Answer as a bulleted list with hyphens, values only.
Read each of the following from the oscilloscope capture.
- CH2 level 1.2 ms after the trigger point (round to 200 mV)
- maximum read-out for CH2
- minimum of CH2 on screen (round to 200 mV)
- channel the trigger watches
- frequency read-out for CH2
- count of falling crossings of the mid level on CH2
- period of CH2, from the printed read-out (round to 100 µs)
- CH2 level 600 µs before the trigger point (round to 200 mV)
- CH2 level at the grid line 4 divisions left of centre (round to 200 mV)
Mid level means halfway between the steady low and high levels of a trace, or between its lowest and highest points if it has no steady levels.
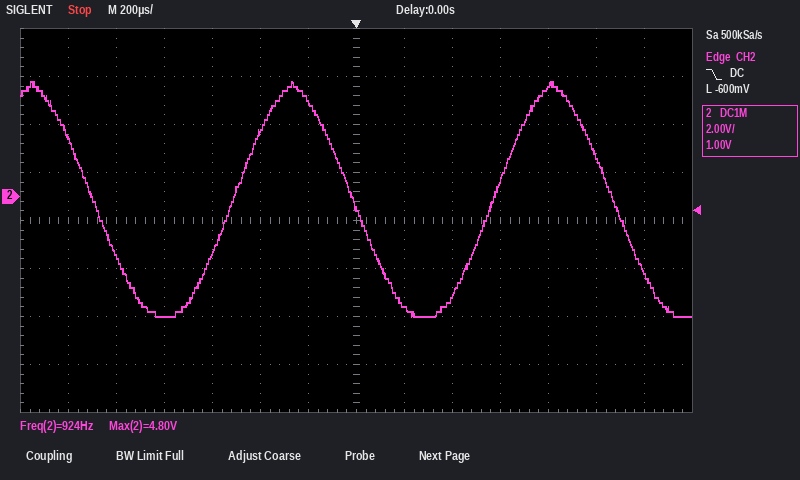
- -3.2 V
- 4.80 V
- -5.0 V
- CH2
- 924 Hz
- 3
- 1.1 ms
- -2.4 V
- -5.0 V
